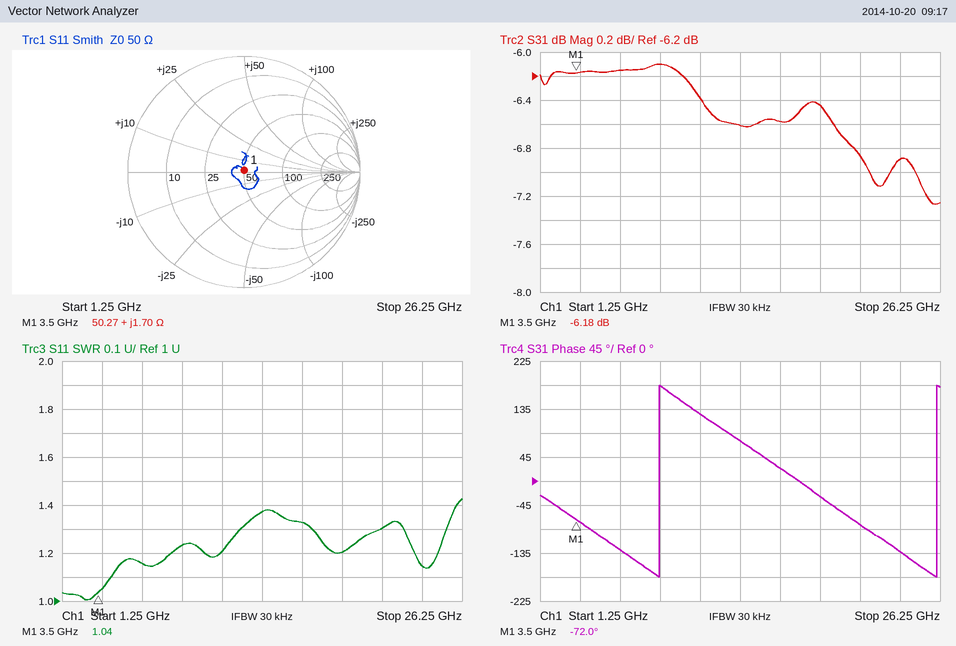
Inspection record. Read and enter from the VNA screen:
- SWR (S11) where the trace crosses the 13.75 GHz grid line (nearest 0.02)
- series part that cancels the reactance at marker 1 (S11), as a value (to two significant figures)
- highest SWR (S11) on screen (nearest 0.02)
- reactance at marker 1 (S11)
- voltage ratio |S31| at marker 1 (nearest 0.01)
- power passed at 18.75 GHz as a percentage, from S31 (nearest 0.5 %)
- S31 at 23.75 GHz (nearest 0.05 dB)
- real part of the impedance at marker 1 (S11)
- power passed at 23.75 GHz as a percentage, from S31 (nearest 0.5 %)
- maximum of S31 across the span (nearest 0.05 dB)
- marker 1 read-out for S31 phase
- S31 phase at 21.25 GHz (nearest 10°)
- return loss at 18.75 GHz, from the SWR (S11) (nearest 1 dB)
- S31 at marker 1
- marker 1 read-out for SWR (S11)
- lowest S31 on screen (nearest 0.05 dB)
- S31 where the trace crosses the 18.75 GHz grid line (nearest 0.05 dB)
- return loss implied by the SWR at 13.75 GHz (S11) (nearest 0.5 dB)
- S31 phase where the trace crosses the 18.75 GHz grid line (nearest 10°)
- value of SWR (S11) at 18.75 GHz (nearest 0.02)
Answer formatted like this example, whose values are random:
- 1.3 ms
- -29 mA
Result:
- 1.38
- 27 pF
- 1.42
- +1.70 Ω
- 0.49
- 22.5 %
- -6.90 dB
- 50.27 Ω
- 20.5 %
- -6.10 dB
- -72.0°
- -80°
- 21 dB
- -6.18 dB
- 1.04
- -7.25 dB
- -6.45 dB
- 16.0 dB
- -30°
- 1.20
